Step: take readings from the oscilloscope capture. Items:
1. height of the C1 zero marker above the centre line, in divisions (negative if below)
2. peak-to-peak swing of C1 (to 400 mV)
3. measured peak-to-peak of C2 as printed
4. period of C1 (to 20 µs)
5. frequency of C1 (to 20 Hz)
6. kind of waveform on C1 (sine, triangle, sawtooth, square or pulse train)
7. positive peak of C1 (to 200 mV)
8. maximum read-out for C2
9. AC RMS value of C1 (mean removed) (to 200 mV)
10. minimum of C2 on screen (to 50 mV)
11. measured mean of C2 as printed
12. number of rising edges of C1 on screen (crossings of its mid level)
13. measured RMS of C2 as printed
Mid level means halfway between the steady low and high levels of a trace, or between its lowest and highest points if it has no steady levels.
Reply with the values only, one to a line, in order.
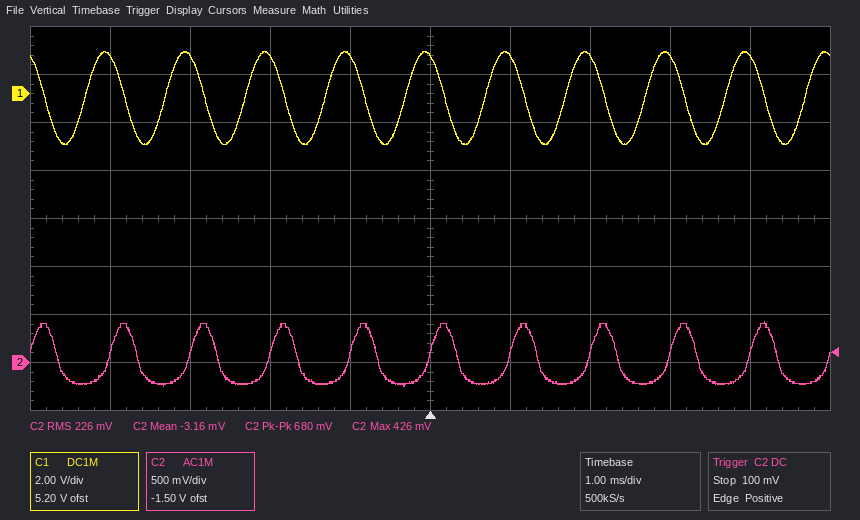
+2.6 div
4.0 V
680 mV
1.00 ms
1.00 kHz
sine
1.8 V
426 mV
1.4 V
-250 mV
-3.16 mV
10
226 mV
